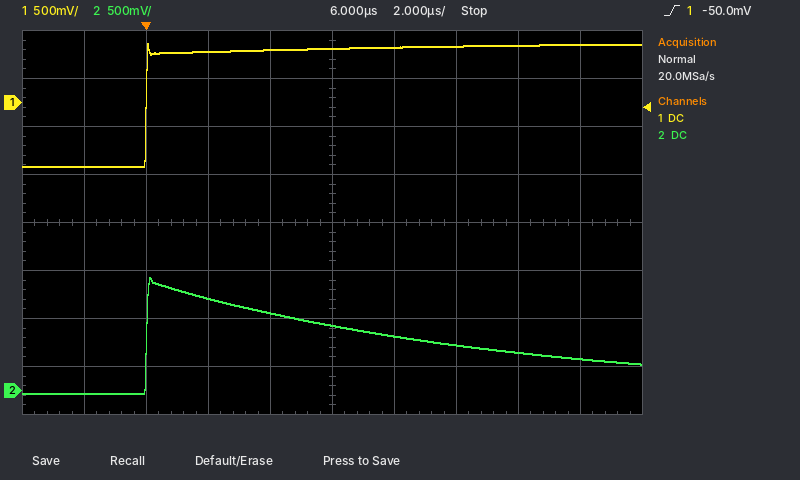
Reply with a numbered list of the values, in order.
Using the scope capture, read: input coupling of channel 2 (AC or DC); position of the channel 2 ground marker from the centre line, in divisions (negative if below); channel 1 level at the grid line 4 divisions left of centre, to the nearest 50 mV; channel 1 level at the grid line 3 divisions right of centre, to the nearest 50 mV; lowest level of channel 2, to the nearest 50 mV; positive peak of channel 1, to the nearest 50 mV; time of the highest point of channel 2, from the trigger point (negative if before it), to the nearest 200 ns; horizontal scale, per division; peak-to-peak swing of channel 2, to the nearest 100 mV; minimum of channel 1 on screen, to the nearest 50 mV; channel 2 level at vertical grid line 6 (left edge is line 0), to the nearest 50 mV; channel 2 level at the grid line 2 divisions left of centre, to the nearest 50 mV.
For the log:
1. DC
2. -3.5 div
3. -650 mV
4. 600 mV
5. -50 mV
6. 600 mV
7. +200 ns
8. 2 µs
9. 1.20 V
10. -650 mV
11. 550 mV
12. 950 mV
